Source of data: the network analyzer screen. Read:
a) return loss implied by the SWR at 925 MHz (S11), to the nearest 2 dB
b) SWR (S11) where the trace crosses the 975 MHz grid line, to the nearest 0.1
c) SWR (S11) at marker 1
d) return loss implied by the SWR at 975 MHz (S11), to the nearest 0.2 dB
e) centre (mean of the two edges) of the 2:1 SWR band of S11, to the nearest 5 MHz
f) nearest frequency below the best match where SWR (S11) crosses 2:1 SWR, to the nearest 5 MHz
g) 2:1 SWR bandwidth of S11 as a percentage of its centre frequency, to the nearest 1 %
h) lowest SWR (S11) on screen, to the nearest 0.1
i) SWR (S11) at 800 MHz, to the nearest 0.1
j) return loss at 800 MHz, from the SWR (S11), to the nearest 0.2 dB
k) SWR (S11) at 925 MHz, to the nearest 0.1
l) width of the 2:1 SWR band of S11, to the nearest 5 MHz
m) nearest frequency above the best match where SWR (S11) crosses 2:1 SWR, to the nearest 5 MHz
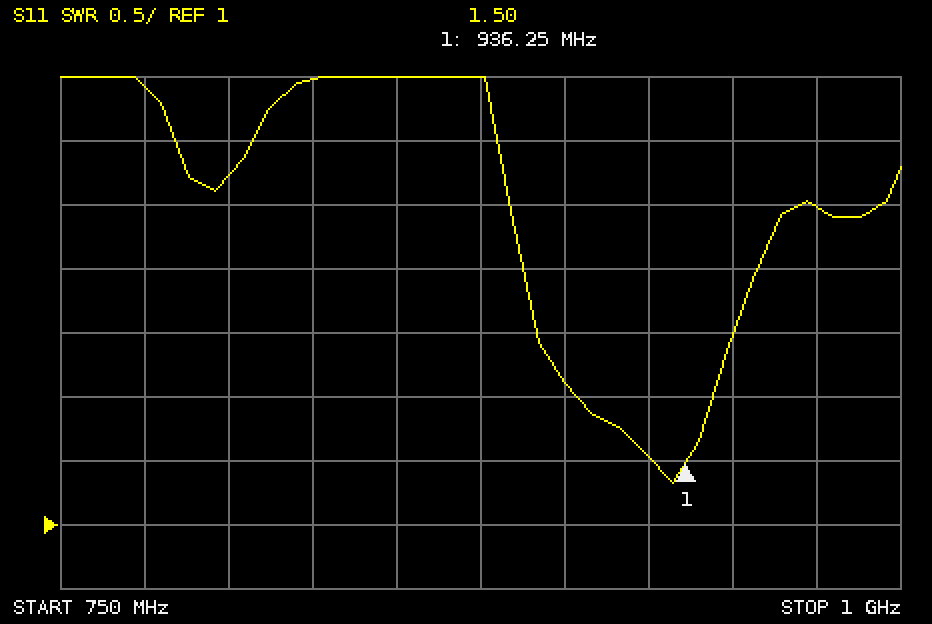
14 dB
3.5
1.50
5.2 dB
925 MHz
905 MHz
4 %
1.3
3.7
4.8 dB
1.5
40 MHz
945 MHz
